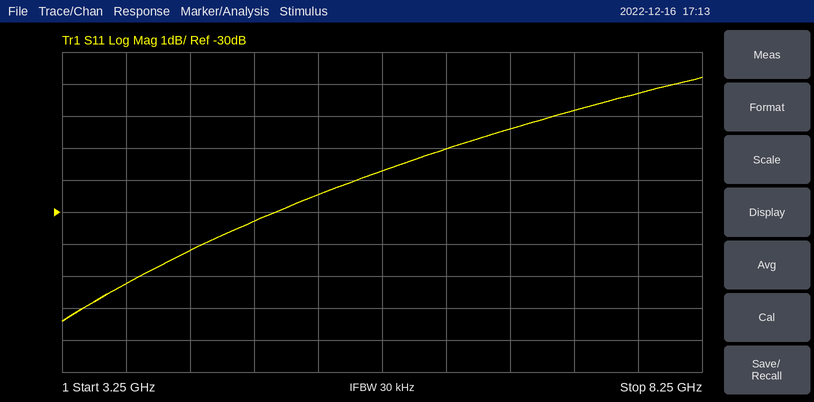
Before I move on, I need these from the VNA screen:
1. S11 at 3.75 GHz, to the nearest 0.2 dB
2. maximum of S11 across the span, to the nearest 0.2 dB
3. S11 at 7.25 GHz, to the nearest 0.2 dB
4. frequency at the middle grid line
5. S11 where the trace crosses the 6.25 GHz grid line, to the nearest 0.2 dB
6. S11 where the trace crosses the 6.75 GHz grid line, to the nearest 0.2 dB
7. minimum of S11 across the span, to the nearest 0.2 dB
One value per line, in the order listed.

-32.2 dB
-25.8 dB
-26.8 dB
5.75 GHz
-28.0 dB
-27.4 dB
-33.4 dB
